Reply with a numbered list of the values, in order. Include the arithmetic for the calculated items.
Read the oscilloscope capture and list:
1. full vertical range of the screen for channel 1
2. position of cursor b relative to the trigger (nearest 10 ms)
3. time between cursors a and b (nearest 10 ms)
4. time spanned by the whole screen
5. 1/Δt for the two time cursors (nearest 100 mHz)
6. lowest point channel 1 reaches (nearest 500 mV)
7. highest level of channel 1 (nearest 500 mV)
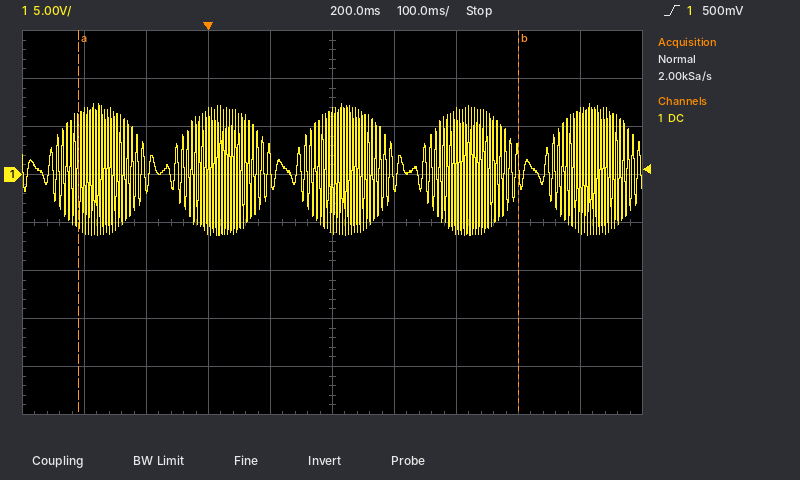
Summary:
1. 40 V
2. +500 ms
3. 710 ms
4. 1 s
5. 1 / 710 ms ≈ 1.4 Hz
6. -6.5 V
7. 7.5 V
